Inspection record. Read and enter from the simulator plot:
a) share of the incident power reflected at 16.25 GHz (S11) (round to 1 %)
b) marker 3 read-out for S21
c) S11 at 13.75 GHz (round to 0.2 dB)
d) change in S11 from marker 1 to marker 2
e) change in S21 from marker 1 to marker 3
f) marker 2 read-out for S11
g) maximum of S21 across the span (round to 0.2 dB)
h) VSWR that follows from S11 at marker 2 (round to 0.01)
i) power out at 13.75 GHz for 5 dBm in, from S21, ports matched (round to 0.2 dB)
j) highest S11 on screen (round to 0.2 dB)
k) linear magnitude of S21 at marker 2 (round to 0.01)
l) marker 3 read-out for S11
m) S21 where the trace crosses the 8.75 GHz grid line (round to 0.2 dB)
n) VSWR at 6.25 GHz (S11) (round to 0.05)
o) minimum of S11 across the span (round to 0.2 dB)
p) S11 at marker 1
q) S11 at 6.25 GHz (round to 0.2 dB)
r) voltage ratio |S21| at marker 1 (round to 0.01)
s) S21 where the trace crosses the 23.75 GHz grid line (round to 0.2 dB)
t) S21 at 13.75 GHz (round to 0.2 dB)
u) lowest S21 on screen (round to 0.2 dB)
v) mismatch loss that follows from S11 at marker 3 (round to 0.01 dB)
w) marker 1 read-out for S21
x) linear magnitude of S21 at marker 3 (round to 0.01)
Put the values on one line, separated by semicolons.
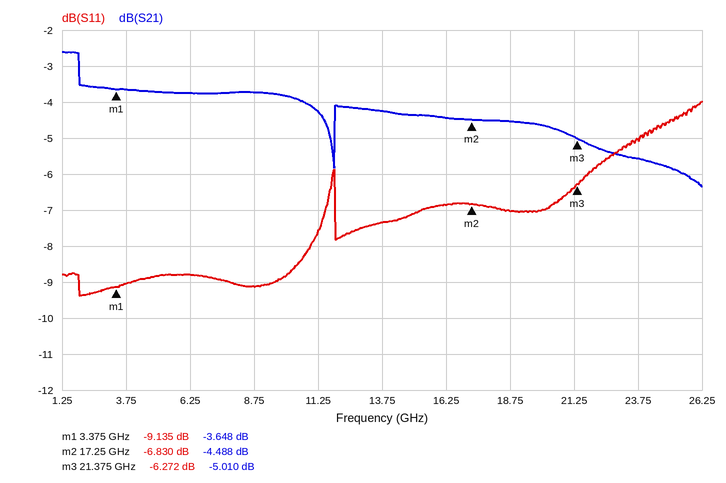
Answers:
21 %; -5.010 dB; -7.4 dB; 2.305 dB; -1.362 dB; -6.830 dB; -2.6 dB; 2.67; 0.8 dBm; -4.0 dB; 0.60; -6.272 dB; -3.8 dB; 2.15; -9.4 dB; -9.135 dB; -8.8 dB; 0.66; -5.6 dB; -4.2 dB; -6.4 dB; 1.17 dB; -3.648 dB; 0.56
